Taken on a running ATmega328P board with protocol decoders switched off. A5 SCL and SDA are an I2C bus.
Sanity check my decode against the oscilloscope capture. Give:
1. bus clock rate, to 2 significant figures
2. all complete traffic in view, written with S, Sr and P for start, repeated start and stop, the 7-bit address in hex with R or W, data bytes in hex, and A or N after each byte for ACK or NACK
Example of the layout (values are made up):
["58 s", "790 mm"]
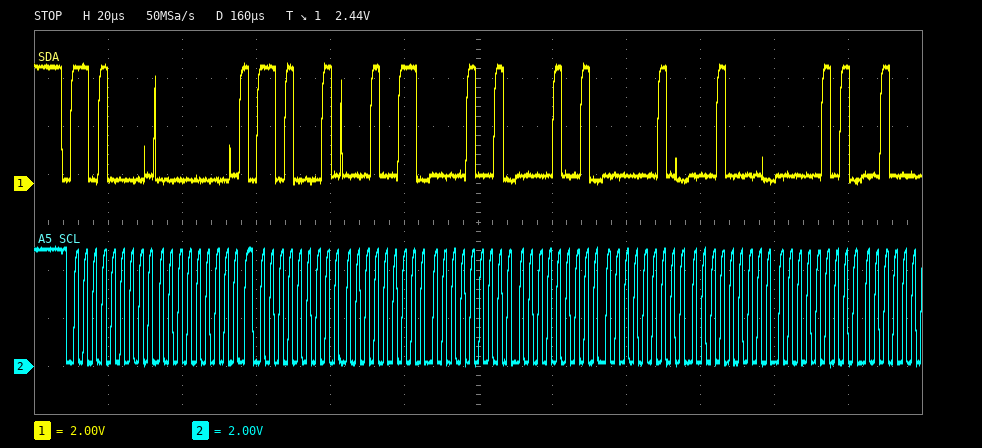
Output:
["400 kHz", "S 68W A 00 A Sr 68R A 13 A 09 A 09 A 02 A 10 A 05 A"]
